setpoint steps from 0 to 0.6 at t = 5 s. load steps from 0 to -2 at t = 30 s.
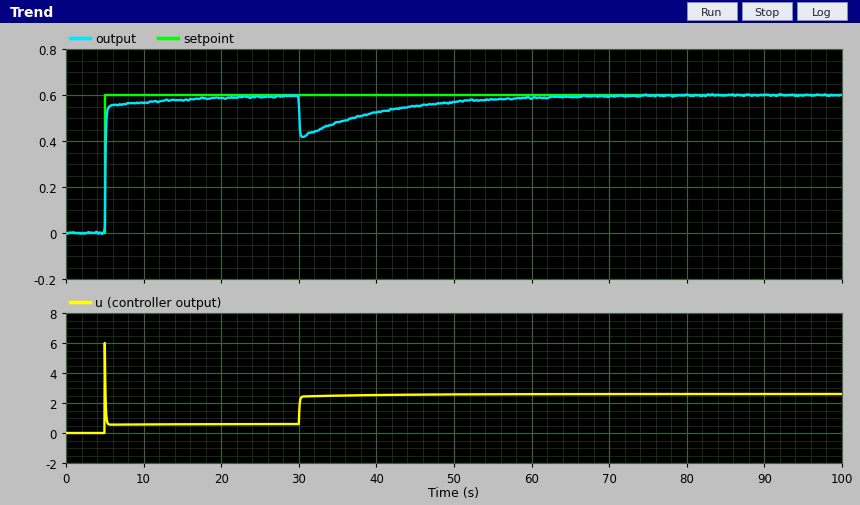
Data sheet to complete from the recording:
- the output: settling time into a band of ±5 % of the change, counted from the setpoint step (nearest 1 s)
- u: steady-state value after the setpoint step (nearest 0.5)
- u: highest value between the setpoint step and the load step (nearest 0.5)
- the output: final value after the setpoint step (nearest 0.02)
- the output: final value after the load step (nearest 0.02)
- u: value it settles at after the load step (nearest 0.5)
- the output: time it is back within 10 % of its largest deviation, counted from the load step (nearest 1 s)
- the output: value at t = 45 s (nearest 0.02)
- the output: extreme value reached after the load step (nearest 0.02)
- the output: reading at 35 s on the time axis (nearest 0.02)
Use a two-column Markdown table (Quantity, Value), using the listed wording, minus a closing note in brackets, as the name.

| Quantity | Value |
|---|---|
| the output: settling time into a band of ±5 % of the change, counted from the setpoint step | 6 s |
| u: steady-state value after the setpoint step | 0.5 |
| u: highest value between the setpoint step and the load step | 6.0 |
| the output: final value after the setpoint step | 0.60 |
| the output: final value after the load step | 0.60 |
| u: value it settles at after the load step | 2.5 |
| the output: time it is back within 10 % of its largest deviation, counted from the load step | 26 s |
| the output: value at t = 45 s | 0.56 |
| the output: extreme value reached after the load step | 0.42 |
| the output: reading at 35 s on the time axis | 0.48 |
